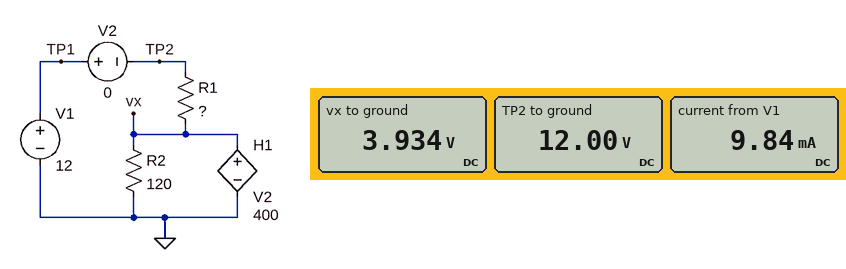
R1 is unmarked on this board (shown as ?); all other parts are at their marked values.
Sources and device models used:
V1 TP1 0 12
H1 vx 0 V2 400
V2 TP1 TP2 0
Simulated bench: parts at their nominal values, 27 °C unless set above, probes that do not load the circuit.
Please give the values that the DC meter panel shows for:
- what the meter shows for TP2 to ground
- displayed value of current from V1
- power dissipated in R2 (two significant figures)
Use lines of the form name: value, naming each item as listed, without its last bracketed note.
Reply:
what the meter shows for TP2 to ground: 12.00 V
displayed value of current from V1: 9.84 mA
power dissipated in R2: 130 mW
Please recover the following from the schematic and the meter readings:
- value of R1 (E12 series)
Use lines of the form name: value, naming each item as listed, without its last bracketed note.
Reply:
value of R1: 820 Ω
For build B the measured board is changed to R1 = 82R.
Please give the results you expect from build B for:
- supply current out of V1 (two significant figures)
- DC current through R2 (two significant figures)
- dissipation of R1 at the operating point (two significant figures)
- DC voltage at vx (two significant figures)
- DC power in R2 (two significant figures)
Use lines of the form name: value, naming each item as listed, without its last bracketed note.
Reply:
supply current out of V1: 25 mA
DC current through R2: 83 mA
dissipation of R1 at the operating point: 51 mW
DC voltage at vx: 10 V
DC power in R2: 830 mW
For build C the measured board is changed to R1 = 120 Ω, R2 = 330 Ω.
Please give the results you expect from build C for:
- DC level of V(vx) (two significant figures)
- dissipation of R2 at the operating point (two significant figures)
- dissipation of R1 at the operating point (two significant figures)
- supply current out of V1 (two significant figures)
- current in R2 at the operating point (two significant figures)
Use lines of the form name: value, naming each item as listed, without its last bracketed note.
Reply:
DC level of V(vx): 9.2 V
dissipation of R2 at the operating point: 260 mW
dissipation of R1 at the operating point: 64 mW
supply current out of V1: 23 mA
current in R2 at the operating point: 28 mA
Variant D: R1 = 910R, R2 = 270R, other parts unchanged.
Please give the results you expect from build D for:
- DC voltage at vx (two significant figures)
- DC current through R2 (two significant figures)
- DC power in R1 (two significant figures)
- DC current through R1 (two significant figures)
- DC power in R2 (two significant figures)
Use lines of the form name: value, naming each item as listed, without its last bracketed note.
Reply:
DC voltage at vx: 3.7 V
DC current through R2: 14 mA
DC power in R1: 76 mW
DC current through R1: 9.2 mA
DC power in R2: 50 mW
